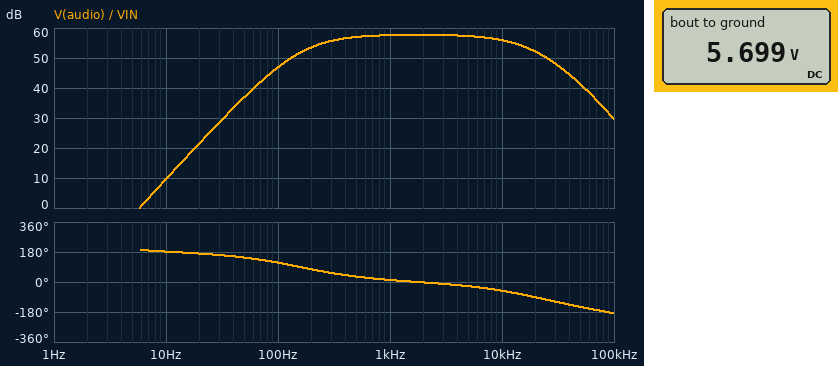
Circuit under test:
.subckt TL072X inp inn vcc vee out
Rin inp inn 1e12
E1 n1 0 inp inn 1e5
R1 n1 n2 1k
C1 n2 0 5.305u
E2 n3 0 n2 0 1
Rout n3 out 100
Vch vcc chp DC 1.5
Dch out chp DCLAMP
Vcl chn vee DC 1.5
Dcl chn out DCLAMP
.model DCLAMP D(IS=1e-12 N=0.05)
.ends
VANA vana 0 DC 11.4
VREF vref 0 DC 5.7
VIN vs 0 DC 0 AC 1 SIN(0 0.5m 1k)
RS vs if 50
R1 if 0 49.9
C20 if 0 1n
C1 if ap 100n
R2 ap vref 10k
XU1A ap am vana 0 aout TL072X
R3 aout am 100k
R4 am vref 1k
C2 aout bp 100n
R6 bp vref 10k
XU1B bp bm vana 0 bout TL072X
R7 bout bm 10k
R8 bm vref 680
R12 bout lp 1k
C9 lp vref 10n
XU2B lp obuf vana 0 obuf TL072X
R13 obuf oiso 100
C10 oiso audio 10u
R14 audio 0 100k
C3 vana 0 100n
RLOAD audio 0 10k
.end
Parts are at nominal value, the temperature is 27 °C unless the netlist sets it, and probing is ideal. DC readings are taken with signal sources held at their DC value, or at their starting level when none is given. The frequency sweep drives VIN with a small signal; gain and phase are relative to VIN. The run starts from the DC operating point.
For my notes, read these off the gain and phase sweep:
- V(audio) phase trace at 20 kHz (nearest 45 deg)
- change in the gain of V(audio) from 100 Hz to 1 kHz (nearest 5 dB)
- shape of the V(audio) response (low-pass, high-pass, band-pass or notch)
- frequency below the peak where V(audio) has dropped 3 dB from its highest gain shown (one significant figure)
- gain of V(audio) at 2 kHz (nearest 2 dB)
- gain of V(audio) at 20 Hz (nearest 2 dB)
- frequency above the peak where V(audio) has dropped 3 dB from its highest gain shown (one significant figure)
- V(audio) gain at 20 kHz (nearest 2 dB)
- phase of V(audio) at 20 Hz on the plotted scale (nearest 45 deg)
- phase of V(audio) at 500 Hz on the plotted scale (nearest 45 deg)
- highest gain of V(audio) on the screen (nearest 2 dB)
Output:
-90 deg
10 dB
band-pass
200 Hz
58 dB
22 dB
10 kHz
52 dB
180 deg
45 deg
58 dB
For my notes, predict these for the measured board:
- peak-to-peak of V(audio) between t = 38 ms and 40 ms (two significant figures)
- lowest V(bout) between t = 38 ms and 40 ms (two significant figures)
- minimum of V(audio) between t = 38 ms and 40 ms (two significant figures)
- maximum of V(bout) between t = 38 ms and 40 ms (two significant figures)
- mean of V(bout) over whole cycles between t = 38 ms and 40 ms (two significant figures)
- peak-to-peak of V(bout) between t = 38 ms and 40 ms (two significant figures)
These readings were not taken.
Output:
760 mV
5.3 V
-380 mV
6.1 V
5.7 V
770 mV
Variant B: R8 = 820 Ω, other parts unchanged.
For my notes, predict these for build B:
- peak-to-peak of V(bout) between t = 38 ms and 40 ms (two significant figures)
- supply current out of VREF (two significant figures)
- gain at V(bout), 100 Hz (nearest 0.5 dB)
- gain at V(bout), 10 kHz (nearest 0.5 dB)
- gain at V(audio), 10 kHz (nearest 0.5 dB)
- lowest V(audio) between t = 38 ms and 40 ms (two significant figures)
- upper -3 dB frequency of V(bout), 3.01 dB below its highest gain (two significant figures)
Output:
650 mV
130 nA
45.5 dB
56.0 dB
54.5 dB
-320 mV
30 kHz
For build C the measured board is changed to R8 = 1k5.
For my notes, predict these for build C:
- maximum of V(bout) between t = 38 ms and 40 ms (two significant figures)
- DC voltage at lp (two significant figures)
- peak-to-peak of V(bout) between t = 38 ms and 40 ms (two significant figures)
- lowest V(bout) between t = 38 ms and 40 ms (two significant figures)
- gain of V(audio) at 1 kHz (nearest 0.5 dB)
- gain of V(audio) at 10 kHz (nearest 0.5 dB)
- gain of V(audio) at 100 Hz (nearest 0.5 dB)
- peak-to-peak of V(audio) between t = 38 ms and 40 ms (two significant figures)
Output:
5.9 V
5.7 V
380 mV
5.5 V
51.5 dB
49.5 dB
40.5 dB
370 mV
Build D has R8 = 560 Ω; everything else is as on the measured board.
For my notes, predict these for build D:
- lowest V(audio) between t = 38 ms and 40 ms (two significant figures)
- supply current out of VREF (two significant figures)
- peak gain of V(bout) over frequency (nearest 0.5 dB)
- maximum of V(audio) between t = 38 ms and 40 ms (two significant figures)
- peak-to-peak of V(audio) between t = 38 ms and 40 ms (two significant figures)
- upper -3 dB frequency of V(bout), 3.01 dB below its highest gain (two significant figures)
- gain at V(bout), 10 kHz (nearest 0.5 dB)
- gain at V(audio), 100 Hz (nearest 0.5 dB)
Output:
-460 mV
160 nA
59.5 dB
460 mV
910 mV
29 kHz
59.0 dB
48.5 dB
